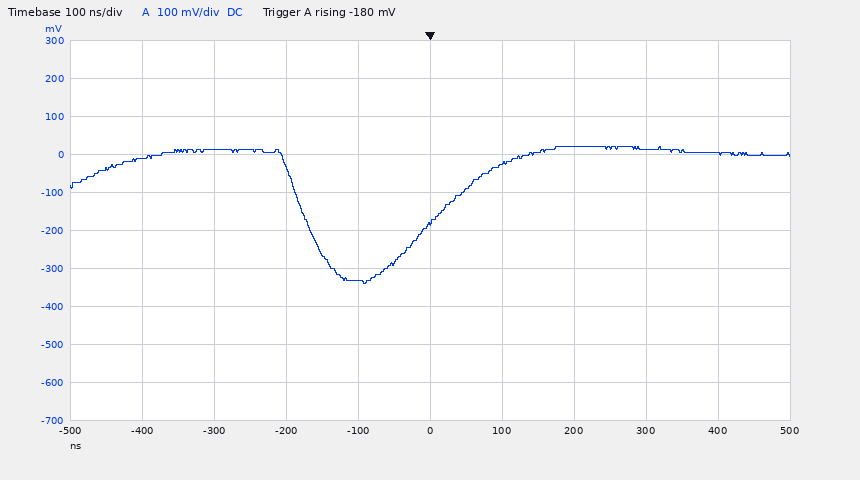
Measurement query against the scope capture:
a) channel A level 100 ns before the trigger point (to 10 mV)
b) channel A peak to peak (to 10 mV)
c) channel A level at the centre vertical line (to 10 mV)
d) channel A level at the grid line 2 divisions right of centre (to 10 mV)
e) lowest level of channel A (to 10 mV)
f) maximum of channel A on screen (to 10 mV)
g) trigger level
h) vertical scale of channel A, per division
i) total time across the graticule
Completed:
-330 mV
360 mV
-180 mV
20 mV
-340 mV
20 mV
-180 mV
100 mV
1 µs
